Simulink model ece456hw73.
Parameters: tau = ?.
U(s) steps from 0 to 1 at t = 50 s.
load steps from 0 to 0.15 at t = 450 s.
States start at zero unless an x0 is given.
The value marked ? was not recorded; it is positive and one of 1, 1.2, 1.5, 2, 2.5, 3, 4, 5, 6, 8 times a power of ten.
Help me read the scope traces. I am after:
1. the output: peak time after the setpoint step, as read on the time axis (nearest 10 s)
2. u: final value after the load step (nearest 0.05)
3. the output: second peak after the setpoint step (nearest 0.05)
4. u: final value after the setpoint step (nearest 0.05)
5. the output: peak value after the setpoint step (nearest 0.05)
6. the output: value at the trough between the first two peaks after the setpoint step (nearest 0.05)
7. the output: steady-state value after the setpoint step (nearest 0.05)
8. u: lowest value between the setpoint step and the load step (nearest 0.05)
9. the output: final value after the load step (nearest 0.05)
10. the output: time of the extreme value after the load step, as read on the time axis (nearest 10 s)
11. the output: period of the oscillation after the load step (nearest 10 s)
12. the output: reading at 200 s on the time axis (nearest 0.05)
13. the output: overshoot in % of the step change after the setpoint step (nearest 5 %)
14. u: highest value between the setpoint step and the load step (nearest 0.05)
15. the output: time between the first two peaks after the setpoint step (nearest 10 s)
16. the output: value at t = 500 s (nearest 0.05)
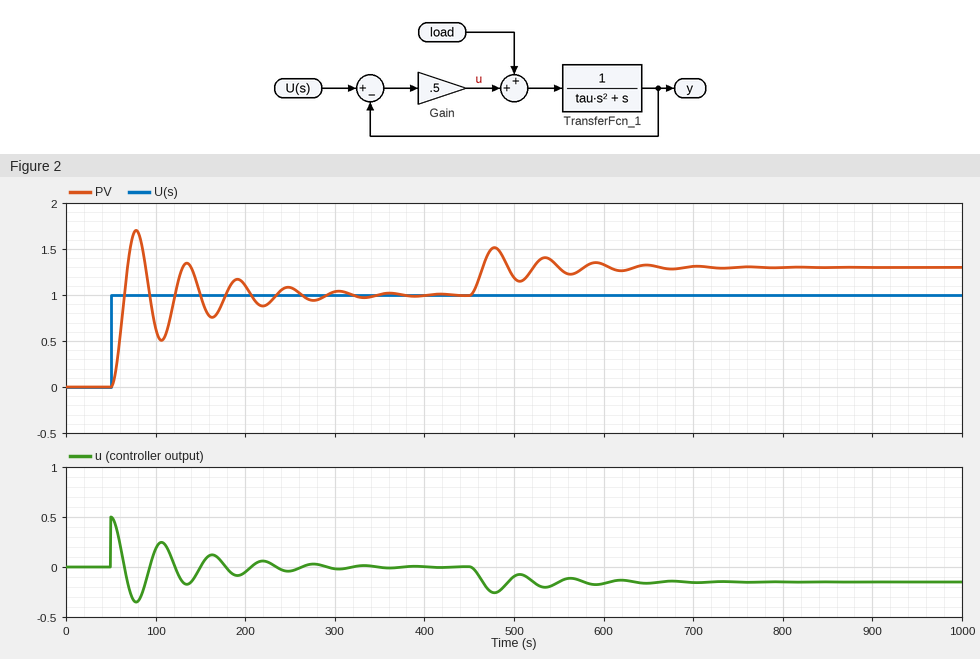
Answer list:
80 s
-0.15
1.35
0.00
1.70
0.50
1.00
-0.35
1.30
480 s
60 s
1.10
70 %
0.50
60 s
1.20
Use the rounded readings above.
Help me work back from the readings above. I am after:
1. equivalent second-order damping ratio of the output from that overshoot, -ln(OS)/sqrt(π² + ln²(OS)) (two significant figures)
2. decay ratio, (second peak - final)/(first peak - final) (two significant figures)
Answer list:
0.11
0.50
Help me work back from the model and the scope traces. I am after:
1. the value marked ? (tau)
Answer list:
40
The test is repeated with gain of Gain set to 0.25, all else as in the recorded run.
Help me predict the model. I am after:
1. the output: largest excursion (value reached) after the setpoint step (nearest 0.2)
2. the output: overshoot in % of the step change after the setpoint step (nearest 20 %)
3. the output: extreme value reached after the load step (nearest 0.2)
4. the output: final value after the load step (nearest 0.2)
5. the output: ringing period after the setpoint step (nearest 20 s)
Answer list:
1.6
60 %
2.0
1.6
80 s
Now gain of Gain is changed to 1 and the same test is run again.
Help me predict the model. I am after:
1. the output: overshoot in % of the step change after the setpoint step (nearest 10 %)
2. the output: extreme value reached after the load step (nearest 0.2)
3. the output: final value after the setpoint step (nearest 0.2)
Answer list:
80 %
1.2
1.0
